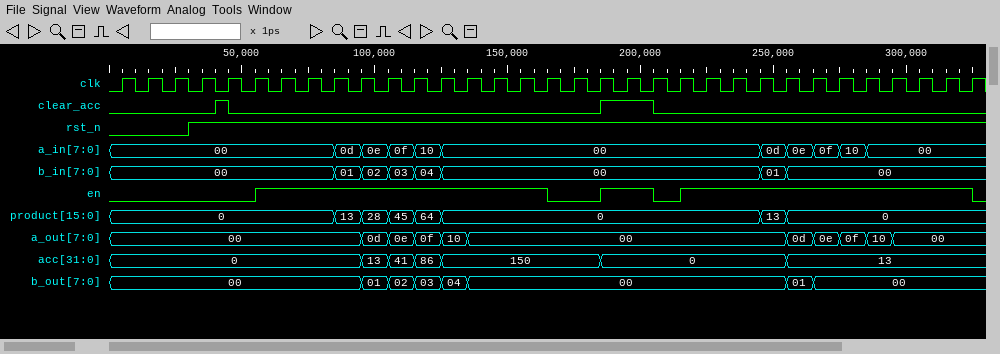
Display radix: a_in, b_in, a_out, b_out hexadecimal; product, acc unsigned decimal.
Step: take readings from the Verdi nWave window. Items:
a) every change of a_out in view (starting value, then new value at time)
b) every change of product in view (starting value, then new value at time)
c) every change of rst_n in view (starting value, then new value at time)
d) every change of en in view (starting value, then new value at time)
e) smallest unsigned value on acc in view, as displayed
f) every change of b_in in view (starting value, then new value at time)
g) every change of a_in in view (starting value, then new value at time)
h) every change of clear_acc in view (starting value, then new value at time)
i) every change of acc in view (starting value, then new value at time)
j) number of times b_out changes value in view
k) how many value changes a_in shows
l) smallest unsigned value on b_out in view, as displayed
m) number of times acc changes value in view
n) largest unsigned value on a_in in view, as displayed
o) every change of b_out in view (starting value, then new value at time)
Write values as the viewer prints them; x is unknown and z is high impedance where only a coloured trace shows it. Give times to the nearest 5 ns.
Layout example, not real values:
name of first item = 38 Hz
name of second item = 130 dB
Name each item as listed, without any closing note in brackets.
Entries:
every change of a_out in view = 00, 0d at 95 ns, 0e at 105 ns, 0f at 115 ns, 10 at 125 ns, 00 at 135 ns, 0d at 255 ns, 0e at 265 ns, 0f at 275 ns, 10 at 285 ns, 00 at 295 ns
every change of product in view = 0, 13 at 85 ns, 28 at 95 ns, 45 at 105 ns, 64 at 115 ns, 0 at 125 ns, 13 at 245 ns, 0 at 255 ns
every change of rst_n in view = 0, 1 at 30 ns
every change of en in view = 0, 1 at 55 ns, 0 at 165 ns, 1 at 185 ns, 0 at 205 ns, 1 at 215 ns, 0 at 325 ns
smallest unsigned value on acc in view, as displayed = 0
every change of b_in in view = 00, 01 at 85 ns, 02 at 95 ns, 03 at 105 ns, 04 at 115 ns, 00 at 125 ns, 01 at 245 ns, 00 at 255 ns
every change of a_in in view = 00, 0d at 85 ns, 0e at 95 ns, 0f at 105 ns, 10 at 115 ns, 00 at 125 ns, 0d at 245 ns, 0e at 255 ns, 0f at 265 ns, 10 at 275 ns, 00 at 285 ns
every change of clear_acc in view = 0, 1 at 40 ns, 0 at 45 ns, 1 at 185 ns, 0 at 205 ns
every change of acc in view = 0, 13 at 95 ns, 41 at 105 ns, 86 at 115 ns, 150 at 125 ns, 0 at 185 ns, 13 at 255 ns
number of times b_out changes value in view = 7
how many value changes a_in shows = 10
smallest unsigned value on b_out in view, as displayed = 00
number of times acc changes value in view = 6
largest unsigned value on a_in in view, as displayed = 10
every change of b_out in view = 00, 01 at 95 ns, 02 at 105 ns, 03 at 115 ns, 04 at 125 ns, 00 at 135 ns, 01 at 255 ns, 00 at 265 ns
